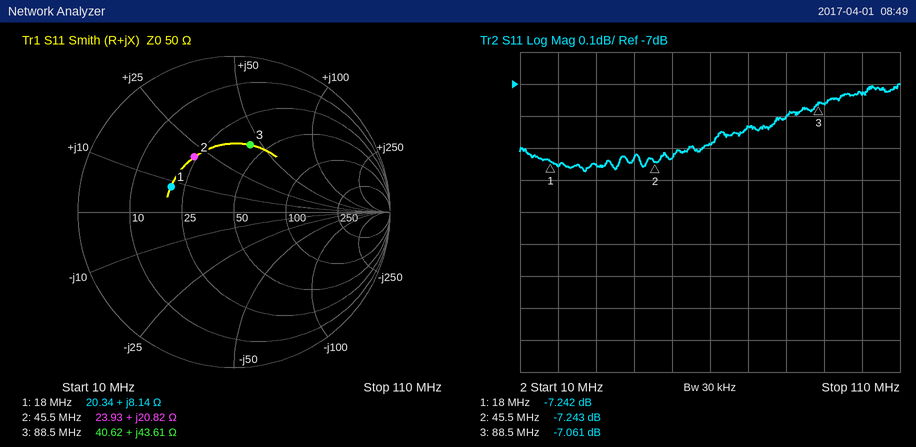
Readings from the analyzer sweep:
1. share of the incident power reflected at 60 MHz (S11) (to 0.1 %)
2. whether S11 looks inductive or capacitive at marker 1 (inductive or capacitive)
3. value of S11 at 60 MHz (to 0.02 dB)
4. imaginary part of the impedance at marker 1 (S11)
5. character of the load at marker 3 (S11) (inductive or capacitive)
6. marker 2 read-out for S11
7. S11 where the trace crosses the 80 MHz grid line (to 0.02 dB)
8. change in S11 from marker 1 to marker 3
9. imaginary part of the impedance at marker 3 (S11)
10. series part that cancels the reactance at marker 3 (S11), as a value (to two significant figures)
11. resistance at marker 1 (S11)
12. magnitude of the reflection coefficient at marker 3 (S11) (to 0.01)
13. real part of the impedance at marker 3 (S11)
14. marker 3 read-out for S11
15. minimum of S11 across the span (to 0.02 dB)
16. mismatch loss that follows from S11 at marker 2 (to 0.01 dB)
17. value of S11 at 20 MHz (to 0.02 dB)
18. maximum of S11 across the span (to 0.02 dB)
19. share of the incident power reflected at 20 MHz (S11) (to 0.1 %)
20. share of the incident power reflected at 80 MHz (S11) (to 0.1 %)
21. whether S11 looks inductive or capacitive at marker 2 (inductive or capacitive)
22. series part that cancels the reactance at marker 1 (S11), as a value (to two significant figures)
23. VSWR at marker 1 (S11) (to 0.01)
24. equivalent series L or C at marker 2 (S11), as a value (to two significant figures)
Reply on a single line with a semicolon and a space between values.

19.1 %; inductive; -7.18 dB; +8.14 Ω; inductive; -7.243 dB; -7.10 dB; 0.181 dB; +43.61 Ω; 41 pF; 20.34 Ω; 0.44; 40.62 Ω; -7.061 dB; -7.28 dB; 0.91 dB; -7.26 dB; -7.00 dB; 18.8 %; 19.5 %; inductive; 1.1 nF; 2.54; 73 nH
